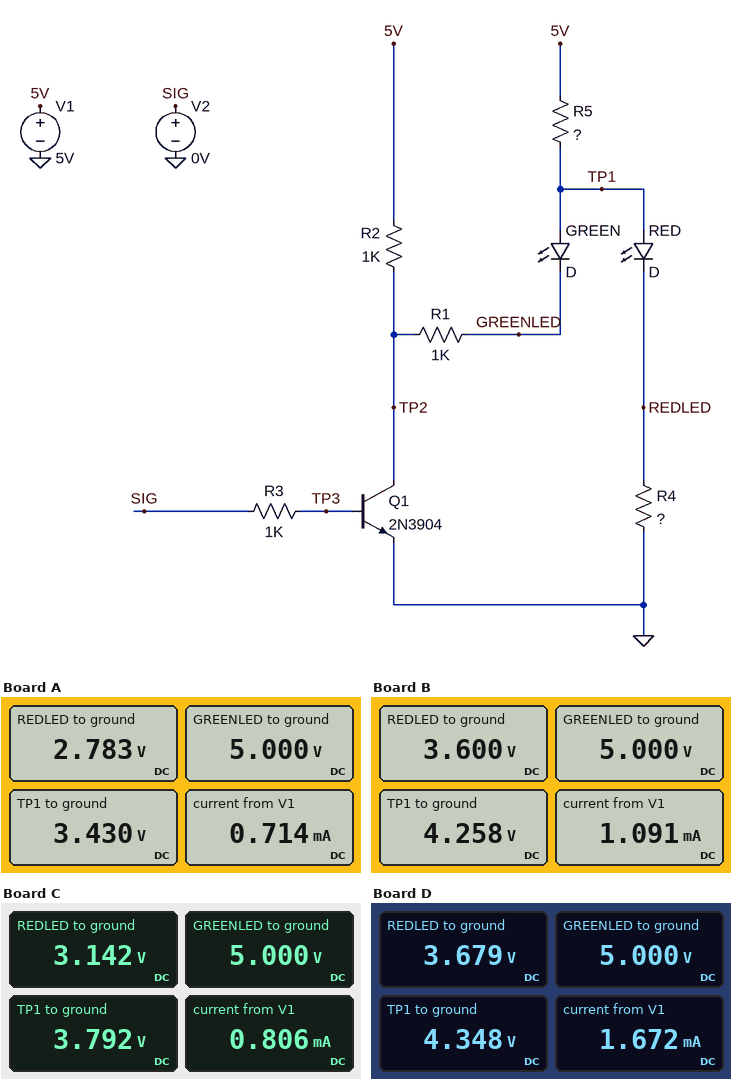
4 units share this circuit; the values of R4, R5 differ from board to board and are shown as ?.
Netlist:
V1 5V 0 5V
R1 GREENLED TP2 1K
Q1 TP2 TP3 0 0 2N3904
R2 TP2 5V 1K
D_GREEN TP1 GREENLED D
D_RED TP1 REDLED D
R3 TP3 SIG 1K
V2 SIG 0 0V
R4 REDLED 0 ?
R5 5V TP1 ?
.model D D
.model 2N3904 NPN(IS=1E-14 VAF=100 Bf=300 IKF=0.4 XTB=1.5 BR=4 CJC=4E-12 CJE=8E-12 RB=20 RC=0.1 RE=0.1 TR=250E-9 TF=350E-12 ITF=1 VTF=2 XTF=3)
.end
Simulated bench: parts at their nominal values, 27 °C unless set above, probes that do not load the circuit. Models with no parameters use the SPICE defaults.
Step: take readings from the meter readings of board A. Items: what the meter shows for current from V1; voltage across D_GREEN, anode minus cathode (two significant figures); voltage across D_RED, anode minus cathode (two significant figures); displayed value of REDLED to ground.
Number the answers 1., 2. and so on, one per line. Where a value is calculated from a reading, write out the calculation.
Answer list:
1. 0.714 mA
2. 3.43 V - 5 V = -1.6 V
3. 3.43 V - 2.783 V = 650 mV
4. 2.783 V
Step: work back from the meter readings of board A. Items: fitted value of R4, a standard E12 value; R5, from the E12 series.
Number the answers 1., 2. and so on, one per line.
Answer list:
1. 3.9 kΩ
2. 2.2 kΩ
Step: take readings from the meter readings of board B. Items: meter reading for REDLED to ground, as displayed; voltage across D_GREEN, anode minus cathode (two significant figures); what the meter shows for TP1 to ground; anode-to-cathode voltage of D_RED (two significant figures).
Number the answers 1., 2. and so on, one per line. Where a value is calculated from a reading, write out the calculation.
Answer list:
1. 3.600 V
2. 4.258 V - 5 V = -740 mV
3. 4.258 V
4. 4.258 V - 3.6 V = 660 mV
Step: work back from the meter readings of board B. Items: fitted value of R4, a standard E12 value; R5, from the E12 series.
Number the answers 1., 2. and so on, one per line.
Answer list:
1. 3.3 kΩ
2. 680 Ω
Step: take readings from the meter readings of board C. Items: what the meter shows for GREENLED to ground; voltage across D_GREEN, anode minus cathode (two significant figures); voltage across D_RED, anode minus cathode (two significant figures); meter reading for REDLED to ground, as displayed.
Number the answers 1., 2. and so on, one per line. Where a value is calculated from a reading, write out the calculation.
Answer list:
1. 5.000 V
2. 3.792 V - 5 V = -1.2 V
3. 3.792 V - 3.142 V = 650 mV
4. 3.142 V
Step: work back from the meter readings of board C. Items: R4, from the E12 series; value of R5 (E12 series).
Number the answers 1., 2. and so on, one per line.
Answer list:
1. 3.9 kΩ
2. 1.5 kΩ
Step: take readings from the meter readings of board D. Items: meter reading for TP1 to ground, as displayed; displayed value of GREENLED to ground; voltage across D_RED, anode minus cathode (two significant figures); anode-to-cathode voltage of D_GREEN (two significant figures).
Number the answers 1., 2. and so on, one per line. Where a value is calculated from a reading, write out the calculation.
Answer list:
1. 4.348 V
2. 5.000 V
3. 4.348 V - 3.679 V = 670 mV
4. 4.348 V - 5 V = -650 mV
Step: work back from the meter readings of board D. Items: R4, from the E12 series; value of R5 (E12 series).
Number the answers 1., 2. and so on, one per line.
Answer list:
1. 2.2 kΩ
2. 390 Ω
